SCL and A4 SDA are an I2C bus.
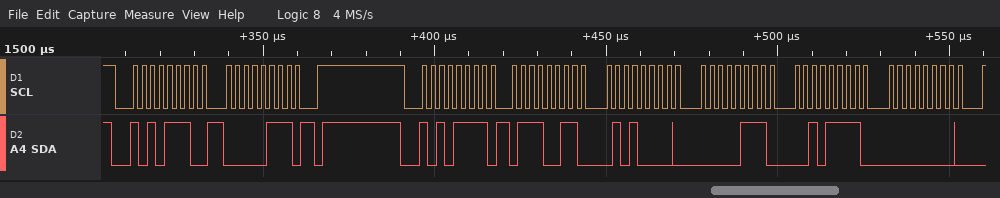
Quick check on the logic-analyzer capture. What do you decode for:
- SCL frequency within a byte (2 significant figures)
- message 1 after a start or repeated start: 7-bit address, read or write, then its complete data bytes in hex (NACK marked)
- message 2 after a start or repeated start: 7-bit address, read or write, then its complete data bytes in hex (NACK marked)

400 kHz
0x57 write: 07
0x57 read: 73 50 07 2F 00
